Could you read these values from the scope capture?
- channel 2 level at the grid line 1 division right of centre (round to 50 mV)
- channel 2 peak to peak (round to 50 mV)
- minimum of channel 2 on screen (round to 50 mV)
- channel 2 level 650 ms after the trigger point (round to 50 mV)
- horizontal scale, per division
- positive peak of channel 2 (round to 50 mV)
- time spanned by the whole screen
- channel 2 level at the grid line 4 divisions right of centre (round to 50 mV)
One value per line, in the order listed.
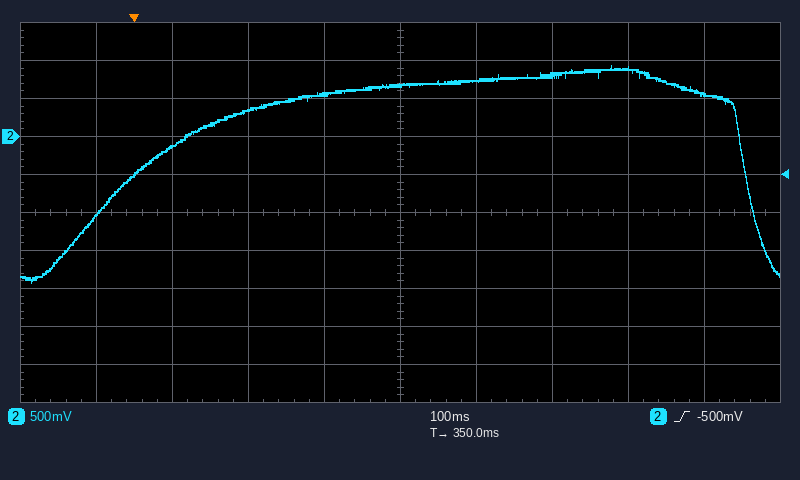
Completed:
750 mV
2.85 V
-1.90 V
900 mV
100 ms
950 mV
1 s
550 mV
